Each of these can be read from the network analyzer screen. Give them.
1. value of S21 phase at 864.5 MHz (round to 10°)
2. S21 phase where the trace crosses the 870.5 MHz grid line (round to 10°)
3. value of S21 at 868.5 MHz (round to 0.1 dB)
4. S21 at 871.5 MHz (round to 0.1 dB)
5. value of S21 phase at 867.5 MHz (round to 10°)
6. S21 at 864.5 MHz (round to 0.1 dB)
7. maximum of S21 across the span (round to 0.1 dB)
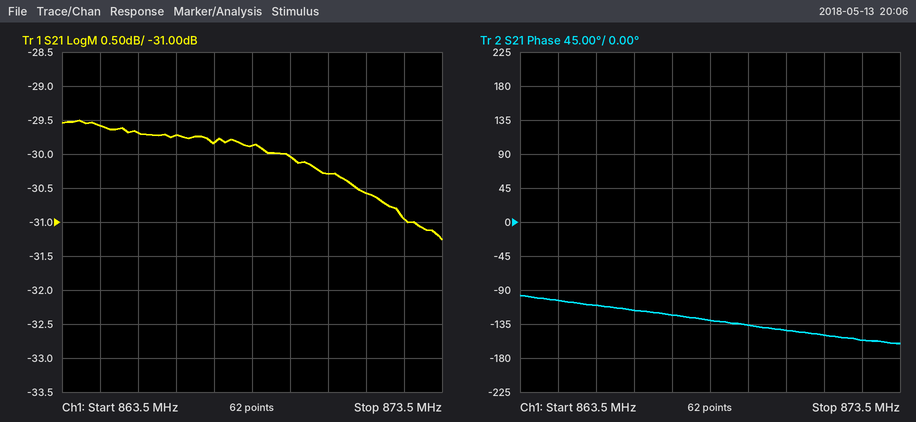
-100°
-140°
-29.9 dB
-30.6 dB
-120°
-29.6 dB
-29.5 dB
